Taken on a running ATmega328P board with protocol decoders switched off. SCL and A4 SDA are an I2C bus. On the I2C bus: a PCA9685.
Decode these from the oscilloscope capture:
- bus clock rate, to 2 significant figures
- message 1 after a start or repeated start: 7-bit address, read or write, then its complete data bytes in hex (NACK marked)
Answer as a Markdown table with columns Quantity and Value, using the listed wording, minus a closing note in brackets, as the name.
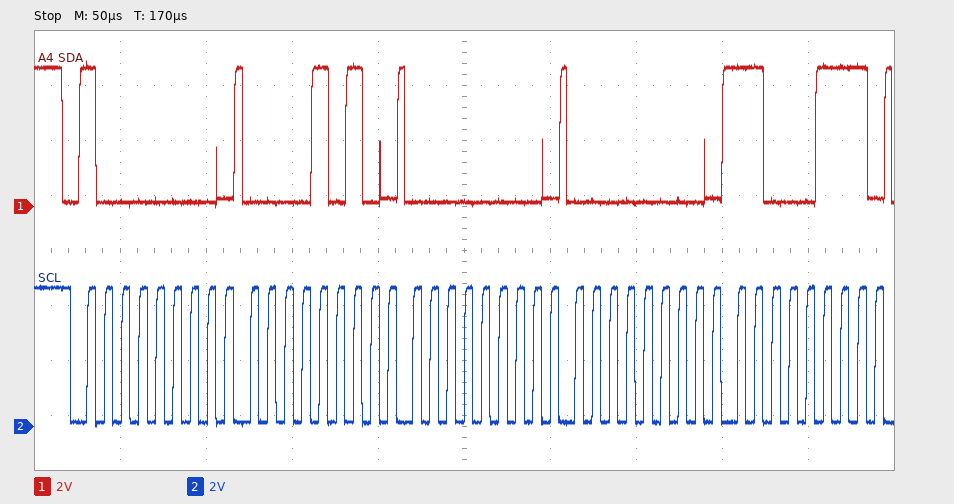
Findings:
| Quantity | Value |
|---|---|
| bus clock rate, to 2 significant figures | 100 kHz |
| message 1 after a start or repeated start: 7-bit address, read or write, then its complete data bytes in hex | 0x40 write: 0A 00 00 C7 |
